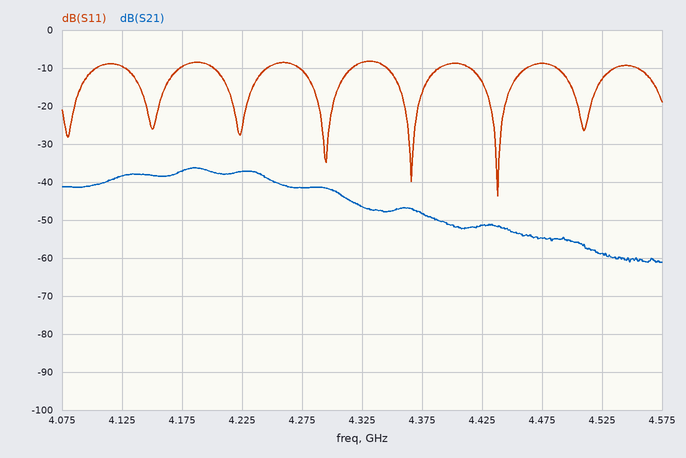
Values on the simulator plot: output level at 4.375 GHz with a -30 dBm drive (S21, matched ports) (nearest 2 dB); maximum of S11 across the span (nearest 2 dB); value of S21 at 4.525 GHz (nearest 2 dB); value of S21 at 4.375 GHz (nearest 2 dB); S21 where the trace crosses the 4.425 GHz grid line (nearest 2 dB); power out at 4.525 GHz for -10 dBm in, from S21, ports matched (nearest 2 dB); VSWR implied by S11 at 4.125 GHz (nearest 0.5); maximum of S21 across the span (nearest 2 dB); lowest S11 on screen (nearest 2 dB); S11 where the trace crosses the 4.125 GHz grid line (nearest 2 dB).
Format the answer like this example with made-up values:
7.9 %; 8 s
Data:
-78 dBm; -8 dB; -58 dB; -48 dB; -52 dB; -68 dBm; 2.0; -36 dB; -44 dB; -10 dB
